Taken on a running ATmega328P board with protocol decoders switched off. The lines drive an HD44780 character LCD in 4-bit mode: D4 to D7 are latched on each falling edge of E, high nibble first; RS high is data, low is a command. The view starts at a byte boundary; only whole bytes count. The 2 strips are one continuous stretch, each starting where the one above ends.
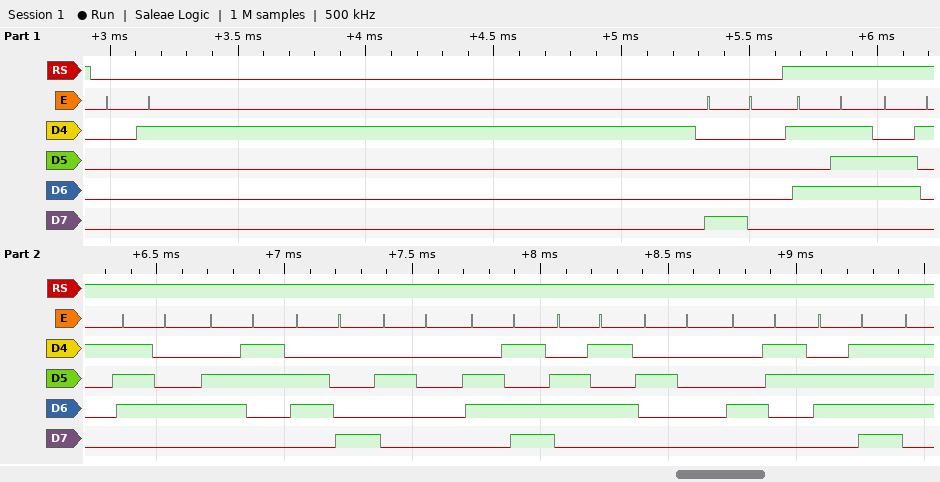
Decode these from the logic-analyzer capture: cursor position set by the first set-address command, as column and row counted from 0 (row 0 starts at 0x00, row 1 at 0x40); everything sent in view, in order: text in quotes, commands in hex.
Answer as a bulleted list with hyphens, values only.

- column 0, row 0
- 0x01 0x80 "Watch me Co"
